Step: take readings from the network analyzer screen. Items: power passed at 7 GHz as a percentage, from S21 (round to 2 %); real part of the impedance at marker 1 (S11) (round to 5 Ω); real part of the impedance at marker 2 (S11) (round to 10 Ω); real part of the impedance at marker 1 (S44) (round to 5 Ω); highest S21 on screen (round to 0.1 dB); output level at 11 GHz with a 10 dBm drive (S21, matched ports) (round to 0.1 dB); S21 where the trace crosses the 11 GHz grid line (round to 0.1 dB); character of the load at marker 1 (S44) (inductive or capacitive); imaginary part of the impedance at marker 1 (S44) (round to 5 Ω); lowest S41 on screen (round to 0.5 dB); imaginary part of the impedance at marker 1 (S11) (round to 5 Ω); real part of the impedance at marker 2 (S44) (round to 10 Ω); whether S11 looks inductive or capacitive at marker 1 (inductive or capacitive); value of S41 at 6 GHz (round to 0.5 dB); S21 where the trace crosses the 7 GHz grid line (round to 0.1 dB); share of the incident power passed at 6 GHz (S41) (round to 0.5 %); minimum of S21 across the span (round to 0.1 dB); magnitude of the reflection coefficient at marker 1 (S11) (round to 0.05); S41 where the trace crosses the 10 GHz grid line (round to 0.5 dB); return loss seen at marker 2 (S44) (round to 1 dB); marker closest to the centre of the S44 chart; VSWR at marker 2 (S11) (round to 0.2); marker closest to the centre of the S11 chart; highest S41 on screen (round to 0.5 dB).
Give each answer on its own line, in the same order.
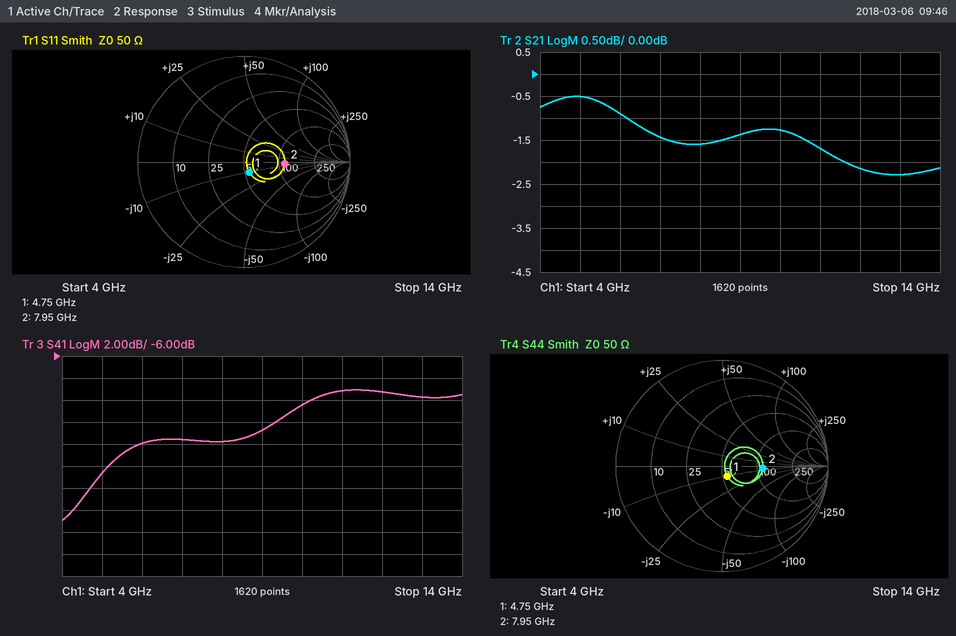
72 %
55 Ω
110 Ω
55 Ω
-0.5 dB
8.3 dBm
-1.7 dB
capacitive
-10 Ω
-21.0 dB
-10 Ω
110 Ω
capacitive
-14.0 dB
-1.4 dB
4.0 %
-2.3 dB
0.10
-10.5 dB
8 dB
marker 1
2.2
marker 1
-9.0 dB
